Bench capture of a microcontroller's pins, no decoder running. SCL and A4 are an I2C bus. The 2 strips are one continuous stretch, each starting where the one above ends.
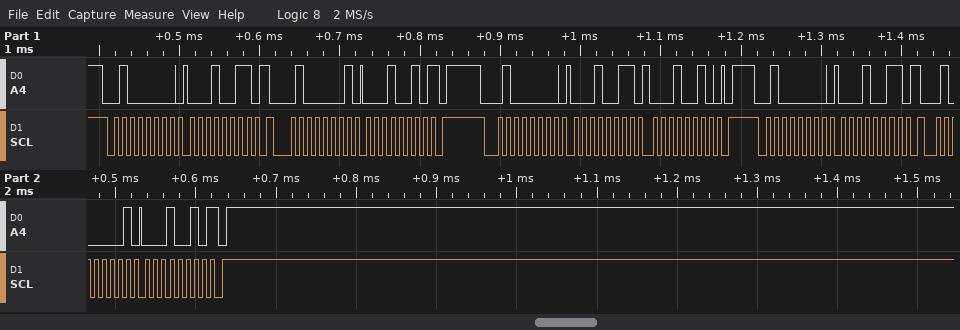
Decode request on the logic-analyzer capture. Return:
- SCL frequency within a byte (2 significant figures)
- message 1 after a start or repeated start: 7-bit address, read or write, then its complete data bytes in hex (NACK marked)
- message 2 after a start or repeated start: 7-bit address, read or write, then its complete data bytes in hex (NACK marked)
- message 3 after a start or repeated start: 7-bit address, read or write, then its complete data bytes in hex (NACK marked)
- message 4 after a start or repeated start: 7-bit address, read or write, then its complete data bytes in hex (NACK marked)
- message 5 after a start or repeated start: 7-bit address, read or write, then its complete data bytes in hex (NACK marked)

100 kHz
0x20 write: 13
0x20 read: 12 NACK
0x20 write: 13 12
0x20 write: 13
0x20 read: 12 NACK
